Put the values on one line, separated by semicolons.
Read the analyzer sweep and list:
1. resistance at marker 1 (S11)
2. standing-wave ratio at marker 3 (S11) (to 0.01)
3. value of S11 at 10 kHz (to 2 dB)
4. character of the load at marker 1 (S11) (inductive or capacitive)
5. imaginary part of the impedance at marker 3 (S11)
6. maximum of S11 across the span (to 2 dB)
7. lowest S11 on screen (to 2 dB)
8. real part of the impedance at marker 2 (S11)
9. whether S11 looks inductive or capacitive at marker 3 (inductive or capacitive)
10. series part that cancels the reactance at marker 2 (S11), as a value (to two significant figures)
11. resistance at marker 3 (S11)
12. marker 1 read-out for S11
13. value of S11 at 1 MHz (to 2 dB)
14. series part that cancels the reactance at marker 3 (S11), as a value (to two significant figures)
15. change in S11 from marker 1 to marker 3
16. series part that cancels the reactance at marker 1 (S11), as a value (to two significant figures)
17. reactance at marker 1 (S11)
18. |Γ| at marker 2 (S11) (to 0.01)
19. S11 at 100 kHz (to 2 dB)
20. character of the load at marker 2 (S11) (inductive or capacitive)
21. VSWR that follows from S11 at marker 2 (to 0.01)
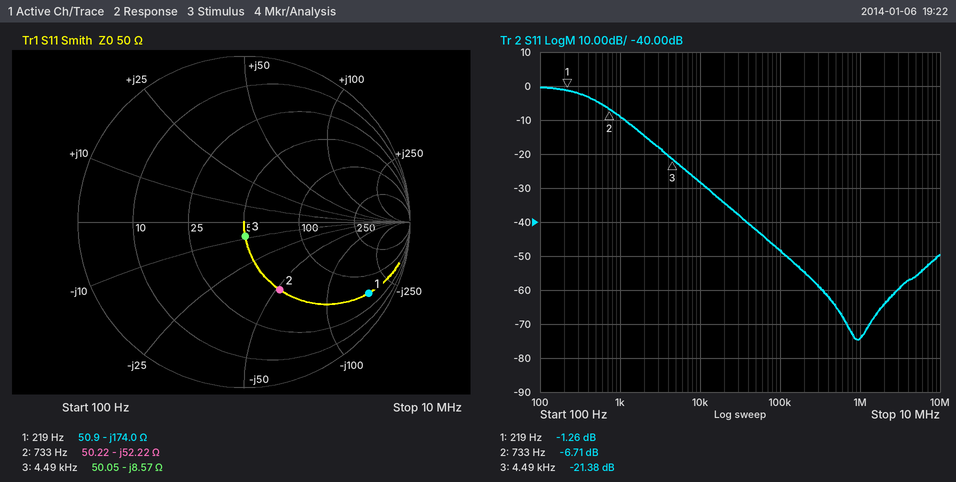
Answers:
50.9 Ω; 1.19; -28 dB; capacitive; -8.57 Ω; 0 dB; -74 dB; 50.22 Ω; capacitive; 11 mH; 50.05 Ω; -1.26 dB; -74 dB; 300 µH; -20.12 dB; 130 mH; -174.0 Ω; 0.46; -48 dB; capacitive; 2.72
